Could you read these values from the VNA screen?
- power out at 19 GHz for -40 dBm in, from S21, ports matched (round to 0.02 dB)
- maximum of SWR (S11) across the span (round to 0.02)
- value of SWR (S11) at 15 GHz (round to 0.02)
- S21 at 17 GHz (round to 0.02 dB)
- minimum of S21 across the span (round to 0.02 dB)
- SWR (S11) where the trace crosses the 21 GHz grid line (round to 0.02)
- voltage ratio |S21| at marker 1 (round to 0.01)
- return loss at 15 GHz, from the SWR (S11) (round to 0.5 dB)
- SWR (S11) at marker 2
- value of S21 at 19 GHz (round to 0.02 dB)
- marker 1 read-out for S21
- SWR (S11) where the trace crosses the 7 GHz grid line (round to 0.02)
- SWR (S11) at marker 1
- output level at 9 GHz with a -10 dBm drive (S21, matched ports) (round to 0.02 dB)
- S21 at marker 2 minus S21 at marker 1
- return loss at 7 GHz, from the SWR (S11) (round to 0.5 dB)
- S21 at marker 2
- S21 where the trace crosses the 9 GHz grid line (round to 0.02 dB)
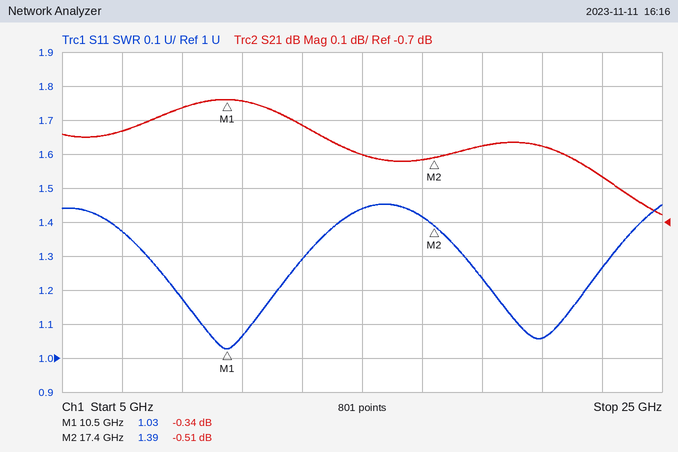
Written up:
-40.48 dBm
1.46
1.44
-0.52 dB
-0.68 dB
1.06
0.96
15.0 dB
1.39
-0.48 dB
-0.34 dB
1.38
1.03
-10.36 dBm
-0.17 dB
16.0 dB
-0.51 dB
-0.36 dB
